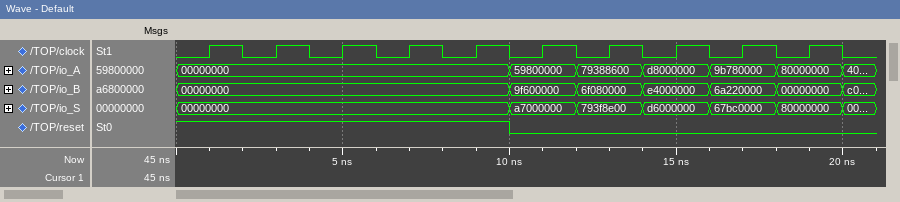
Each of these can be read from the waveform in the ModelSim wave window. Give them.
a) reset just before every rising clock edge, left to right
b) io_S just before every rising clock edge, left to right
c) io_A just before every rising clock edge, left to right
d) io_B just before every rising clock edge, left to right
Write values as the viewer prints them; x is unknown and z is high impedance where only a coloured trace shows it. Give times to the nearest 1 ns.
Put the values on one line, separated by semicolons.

1 1 1 1 1 0 0 0 0 0; 00000000, 00000000, 00000000, 00000000, 00000000, a7000000, 793f8e00, d6000000, 67bc0000, 80000000; 00000000, 00000000, 00000000, 00000000, 00000000, 59800000, 79388600, d8000000, 9b780000, 80000000; 00000000, 00000000, 00000000, 00000000, 00000000, 9f600000, 6f080000, e4000000, 6a220000, 00000000
